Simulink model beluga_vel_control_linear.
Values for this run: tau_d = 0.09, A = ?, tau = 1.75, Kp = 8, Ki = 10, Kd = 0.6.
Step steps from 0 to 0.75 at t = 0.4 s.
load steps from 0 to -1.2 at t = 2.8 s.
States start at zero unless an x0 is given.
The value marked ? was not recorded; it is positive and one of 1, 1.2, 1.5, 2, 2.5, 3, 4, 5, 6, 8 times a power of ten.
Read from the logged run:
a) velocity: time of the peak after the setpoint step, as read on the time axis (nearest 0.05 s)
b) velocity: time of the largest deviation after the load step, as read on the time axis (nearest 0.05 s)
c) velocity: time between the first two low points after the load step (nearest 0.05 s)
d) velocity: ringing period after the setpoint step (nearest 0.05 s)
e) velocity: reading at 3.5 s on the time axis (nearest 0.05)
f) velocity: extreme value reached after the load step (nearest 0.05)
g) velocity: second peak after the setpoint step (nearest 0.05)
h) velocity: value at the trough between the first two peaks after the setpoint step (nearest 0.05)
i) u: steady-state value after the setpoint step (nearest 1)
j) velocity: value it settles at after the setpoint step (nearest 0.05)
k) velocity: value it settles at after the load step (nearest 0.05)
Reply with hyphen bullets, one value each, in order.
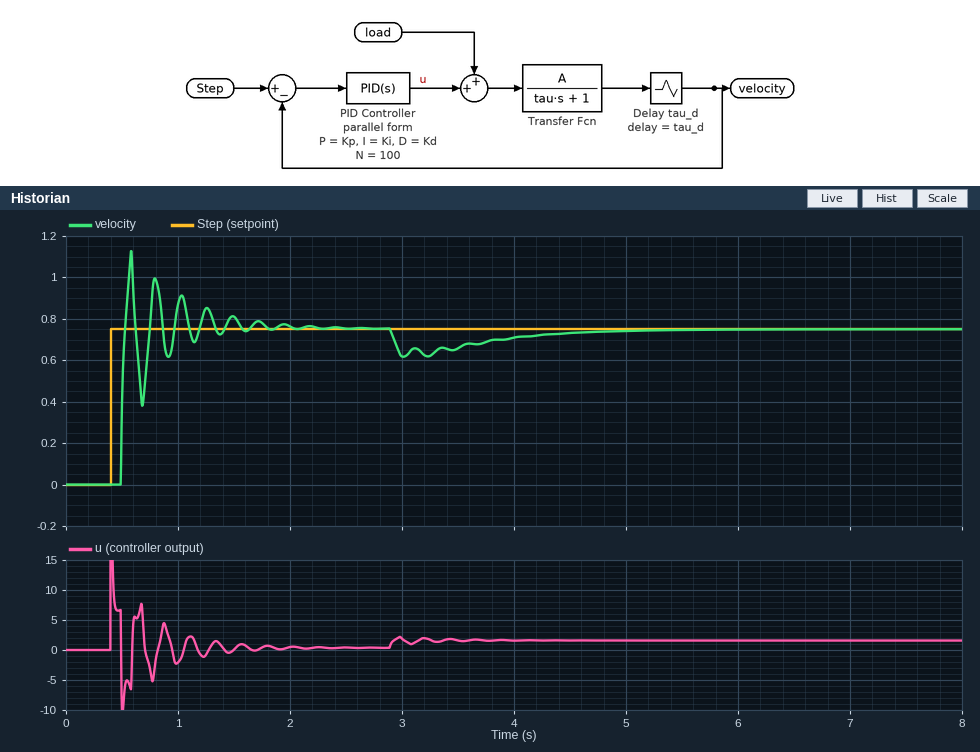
- 0.60 s
- 3.00 s
- 0.20 s
- 0.20 s
- 0.65
- 0.60
- 1.00
- 0.40
- 0
- 0.75
- 0.75
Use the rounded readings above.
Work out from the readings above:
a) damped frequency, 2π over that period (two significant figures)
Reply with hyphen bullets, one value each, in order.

- 31 rad/s
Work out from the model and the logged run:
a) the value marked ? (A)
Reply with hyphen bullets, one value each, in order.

- 2
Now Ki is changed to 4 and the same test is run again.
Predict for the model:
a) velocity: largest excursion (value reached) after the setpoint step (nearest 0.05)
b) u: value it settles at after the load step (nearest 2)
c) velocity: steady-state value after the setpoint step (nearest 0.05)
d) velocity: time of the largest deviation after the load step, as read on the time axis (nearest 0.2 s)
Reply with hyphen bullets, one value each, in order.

- 1.10
- 2
- 0.75
- 3.2 s
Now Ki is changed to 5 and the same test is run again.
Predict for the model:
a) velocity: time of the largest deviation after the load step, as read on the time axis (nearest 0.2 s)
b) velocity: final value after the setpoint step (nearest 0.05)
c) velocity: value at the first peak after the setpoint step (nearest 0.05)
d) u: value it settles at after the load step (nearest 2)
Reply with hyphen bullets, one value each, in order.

- 3.2 s
- 0.75
- 1.10
- 2
